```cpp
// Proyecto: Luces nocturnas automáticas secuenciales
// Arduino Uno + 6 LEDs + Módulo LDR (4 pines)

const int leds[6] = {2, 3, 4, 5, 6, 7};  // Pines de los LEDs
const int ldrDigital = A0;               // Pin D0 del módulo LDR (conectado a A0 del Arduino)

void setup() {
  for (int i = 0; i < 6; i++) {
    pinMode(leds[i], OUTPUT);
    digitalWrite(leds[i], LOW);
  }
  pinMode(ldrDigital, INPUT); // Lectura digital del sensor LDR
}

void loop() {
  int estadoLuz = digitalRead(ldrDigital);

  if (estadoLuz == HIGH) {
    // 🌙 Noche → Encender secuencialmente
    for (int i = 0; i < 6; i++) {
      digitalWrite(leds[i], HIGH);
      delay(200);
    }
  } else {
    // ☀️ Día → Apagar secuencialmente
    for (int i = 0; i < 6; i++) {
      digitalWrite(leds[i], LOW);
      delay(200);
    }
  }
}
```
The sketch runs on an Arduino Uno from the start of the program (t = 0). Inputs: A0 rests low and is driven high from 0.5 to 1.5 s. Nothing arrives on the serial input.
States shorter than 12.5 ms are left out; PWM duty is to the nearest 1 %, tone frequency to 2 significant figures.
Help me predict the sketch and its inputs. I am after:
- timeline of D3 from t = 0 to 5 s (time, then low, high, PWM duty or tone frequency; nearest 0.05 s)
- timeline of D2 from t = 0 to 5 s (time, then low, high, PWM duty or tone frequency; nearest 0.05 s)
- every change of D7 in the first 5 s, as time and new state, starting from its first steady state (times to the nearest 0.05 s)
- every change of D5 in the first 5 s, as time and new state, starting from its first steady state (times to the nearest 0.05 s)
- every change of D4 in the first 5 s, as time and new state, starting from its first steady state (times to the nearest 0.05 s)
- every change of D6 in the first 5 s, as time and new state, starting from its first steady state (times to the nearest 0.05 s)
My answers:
0 s low; 1.4 s high; 2.6 s low
0 s low; 1.2 s high; 2.4 s low
0 s low; 2.2 s high; 3.4 s low
0 s low; 1.8 s high; 3 s low
0 s low; 1.6 s high; 2.8 s low
0 s low; 2 s high; 3.2 s low
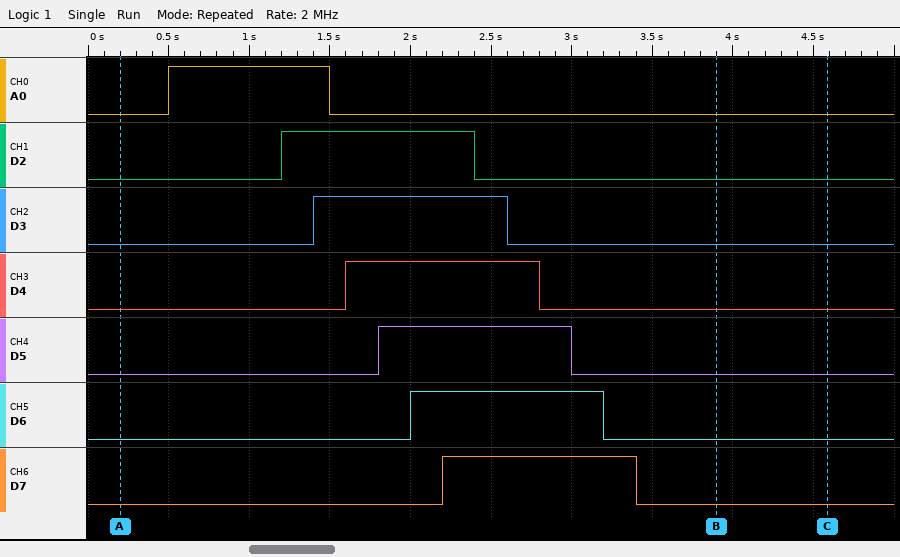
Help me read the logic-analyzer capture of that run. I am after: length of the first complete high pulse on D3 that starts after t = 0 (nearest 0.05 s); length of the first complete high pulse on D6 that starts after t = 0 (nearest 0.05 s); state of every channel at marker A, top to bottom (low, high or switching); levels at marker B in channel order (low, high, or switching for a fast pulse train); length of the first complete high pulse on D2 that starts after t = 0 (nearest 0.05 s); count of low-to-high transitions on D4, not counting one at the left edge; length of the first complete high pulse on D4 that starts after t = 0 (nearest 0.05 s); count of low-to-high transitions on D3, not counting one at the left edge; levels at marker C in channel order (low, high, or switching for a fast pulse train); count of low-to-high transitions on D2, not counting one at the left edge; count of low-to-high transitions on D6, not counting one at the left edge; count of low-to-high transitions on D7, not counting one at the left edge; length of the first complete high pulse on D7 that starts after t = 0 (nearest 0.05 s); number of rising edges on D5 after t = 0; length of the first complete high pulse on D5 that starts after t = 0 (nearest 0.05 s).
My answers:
1.20 s
1.20 s
A0 low, D2 low, D3 low, D4 low, D5 low, D6 low, D7 low
A0 low, D2 low, D3 low, D4 low, D5 low, D6 low, D7 low
1.20 s
1
1.20 s
1
A0 low, D2 low, D3 low, D4 low, D5 low, D6 low, D7 low
1
1
1
1.20 s
1
1.20 s
